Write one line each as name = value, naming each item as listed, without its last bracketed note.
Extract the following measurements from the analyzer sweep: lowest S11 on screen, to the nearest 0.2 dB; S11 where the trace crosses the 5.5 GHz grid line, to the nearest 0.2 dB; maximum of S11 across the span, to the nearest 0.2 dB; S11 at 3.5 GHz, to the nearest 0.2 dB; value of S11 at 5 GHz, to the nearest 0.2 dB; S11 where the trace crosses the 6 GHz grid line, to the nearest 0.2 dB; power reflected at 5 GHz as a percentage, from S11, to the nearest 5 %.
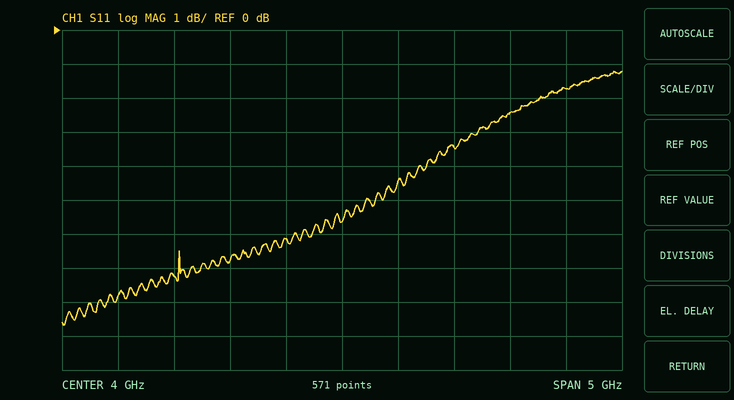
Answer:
lowest S11 on screen, to the nearest 0.2 dB = -8.6 dB
S11 where the trace crosses the 5.5 GHz grid line, to the nearest 0.2 dB = -2.4 dB
maximum of S11 across the span, to the nearest 0.2 dB = -1.2 dB
S11 at 3.5 GHz, to the nearest 0.2 dB = -6.2 dB
value of S11 at 5 GHz, to the nearest 0.2 dB = -3.4 dB
S11 where the trace crosses the 6 GHz grid line, to the nearest 0.2 dB = -1.8 dB
power reflected at 5 GHz as a percentage, from S11, to the nearest 5 % = 45 %
